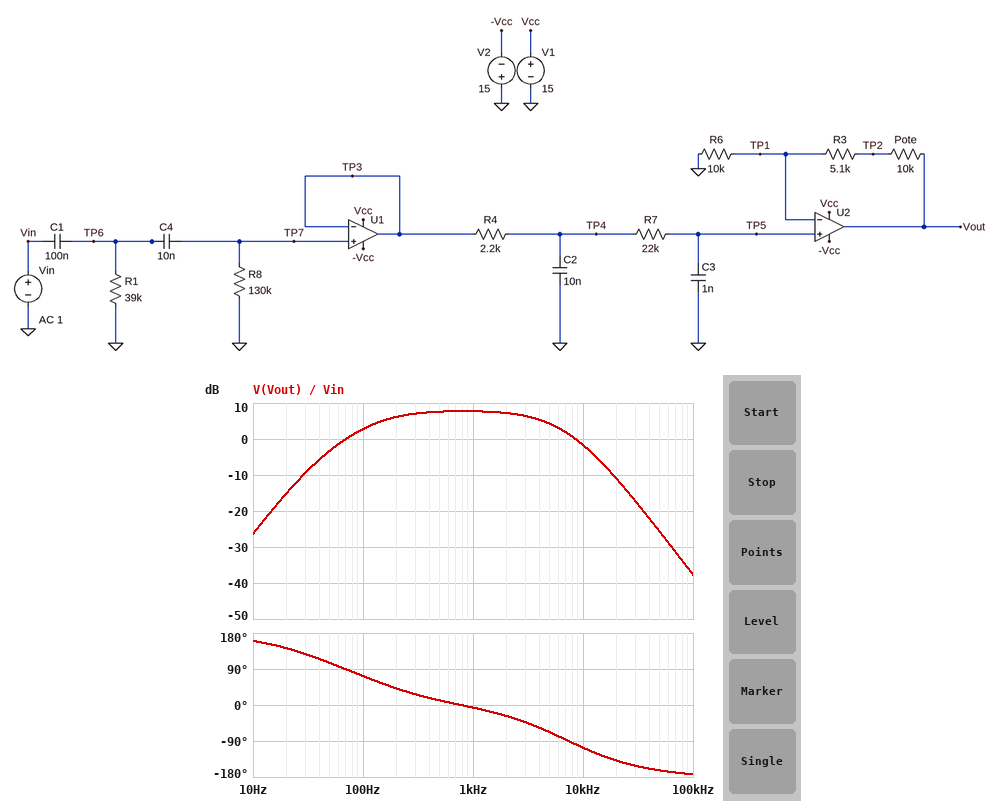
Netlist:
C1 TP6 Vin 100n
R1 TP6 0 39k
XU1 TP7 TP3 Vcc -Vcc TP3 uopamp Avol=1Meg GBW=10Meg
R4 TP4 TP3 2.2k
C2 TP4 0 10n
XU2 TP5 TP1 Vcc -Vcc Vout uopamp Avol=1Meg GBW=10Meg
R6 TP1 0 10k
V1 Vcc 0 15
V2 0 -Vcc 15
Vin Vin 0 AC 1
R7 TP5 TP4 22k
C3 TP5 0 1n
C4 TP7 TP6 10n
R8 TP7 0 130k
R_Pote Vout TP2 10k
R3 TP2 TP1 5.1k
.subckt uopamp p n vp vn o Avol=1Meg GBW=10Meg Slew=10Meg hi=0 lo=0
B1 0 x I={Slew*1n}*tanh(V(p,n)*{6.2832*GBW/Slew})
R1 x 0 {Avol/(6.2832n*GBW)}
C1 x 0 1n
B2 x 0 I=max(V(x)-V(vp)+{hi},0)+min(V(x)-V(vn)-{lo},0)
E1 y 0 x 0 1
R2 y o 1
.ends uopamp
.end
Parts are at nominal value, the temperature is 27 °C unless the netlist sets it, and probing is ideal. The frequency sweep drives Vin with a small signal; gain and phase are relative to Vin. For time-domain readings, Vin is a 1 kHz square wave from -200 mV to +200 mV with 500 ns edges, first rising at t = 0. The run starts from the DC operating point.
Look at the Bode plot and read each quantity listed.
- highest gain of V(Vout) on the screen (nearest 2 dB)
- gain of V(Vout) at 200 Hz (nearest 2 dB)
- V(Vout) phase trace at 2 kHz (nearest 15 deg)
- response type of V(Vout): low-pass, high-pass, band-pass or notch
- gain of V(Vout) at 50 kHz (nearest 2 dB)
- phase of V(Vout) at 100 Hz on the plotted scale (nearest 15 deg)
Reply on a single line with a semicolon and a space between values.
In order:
8 dB; 6 dB; -30 deg; band-pass; -26 dB; 75 deg
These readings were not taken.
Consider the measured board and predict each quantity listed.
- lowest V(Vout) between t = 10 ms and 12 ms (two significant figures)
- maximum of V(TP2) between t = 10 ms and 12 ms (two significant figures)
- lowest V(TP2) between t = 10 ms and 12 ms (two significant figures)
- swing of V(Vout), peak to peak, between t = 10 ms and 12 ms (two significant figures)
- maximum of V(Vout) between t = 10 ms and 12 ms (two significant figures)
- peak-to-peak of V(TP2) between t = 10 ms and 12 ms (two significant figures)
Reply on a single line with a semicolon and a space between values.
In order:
-570 mV; 330 mV; -340 mV; 1.1 V; 540 mV; 670 mV
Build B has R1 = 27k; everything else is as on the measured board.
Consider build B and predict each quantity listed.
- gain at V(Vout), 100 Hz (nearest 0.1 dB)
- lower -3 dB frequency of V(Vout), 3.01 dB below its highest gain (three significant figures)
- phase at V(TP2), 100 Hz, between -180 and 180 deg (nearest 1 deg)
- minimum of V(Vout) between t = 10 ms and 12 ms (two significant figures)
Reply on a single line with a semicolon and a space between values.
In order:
2.2 dB; 150 Hz; 80 deg; -570 mV
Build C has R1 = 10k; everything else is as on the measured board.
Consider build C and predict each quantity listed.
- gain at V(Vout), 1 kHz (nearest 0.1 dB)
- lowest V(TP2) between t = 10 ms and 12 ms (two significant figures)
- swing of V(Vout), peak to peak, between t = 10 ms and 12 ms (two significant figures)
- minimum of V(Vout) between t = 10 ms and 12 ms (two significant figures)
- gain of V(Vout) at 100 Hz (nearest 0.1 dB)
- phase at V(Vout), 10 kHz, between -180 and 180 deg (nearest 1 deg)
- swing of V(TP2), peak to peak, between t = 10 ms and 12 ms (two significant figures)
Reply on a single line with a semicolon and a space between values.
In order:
7.6 dB; -360 mV; 1.2 V; -600 mV; -1.8 dB; -106 deg; 720 mV
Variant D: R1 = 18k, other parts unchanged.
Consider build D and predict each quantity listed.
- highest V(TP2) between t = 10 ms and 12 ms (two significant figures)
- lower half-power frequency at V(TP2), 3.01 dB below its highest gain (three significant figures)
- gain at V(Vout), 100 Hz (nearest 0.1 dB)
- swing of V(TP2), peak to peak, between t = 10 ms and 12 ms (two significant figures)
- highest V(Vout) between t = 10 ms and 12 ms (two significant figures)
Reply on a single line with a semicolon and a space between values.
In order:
340 mV; 168 Hz; 1.0 dB; 690 mV; 570 mV
